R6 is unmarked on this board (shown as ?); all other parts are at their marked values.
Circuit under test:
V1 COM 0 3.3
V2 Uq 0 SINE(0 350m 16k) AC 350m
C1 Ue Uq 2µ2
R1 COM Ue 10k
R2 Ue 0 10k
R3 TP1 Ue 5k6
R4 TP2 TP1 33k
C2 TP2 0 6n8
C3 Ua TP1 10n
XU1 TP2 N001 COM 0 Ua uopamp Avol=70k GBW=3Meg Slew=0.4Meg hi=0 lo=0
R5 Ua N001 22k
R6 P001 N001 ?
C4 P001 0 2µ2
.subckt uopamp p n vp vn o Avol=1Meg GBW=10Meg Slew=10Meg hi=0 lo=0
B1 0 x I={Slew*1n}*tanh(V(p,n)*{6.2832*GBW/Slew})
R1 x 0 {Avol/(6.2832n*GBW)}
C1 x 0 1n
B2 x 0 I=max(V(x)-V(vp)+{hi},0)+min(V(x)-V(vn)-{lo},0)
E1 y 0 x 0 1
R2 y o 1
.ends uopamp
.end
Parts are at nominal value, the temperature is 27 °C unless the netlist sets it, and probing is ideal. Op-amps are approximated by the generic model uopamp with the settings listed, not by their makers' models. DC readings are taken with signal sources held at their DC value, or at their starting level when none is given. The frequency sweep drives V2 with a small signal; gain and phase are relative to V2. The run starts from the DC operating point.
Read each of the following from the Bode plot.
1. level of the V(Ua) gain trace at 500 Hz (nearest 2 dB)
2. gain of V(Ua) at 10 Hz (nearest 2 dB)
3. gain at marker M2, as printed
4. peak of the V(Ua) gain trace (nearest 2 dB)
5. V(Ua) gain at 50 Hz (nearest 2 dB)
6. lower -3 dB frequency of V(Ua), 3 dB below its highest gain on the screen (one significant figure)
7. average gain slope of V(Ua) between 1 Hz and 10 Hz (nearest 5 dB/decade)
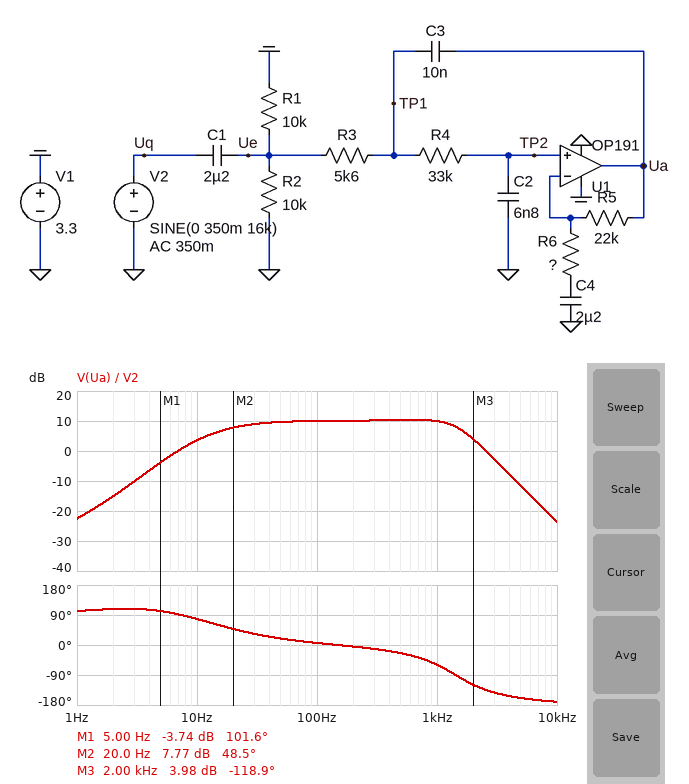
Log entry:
10 dB
4 dB
7.77 dB
10 dB
10 dB
20 Hz
25 dB/decade
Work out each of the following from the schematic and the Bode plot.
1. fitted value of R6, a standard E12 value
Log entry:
10 kΩ
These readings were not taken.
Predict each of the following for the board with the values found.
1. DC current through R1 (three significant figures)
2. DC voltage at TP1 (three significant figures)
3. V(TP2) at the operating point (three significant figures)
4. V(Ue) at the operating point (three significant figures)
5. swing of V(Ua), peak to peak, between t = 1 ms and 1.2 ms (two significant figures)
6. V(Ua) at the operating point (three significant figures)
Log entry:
165 µA
1.65 V
1.65 V
1.65 V
18 mV
1.65 V
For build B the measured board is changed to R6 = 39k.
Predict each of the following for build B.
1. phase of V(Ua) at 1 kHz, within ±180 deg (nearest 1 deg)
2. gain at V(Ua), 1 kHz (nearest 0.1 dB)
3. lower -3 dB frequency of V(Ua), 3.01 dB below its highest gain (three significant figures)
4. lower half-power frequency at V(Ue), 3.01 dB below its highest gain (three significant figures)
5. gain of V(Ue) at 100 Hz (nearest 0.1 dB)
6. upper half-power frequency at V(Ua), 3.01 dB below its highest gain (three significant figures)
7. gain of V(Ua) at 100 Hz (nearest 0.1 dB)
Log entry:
-70 deg
0.1 dB
14.2 Hz
14.5 Hz
-0.1 dB
895 Hz
3.7 dB
